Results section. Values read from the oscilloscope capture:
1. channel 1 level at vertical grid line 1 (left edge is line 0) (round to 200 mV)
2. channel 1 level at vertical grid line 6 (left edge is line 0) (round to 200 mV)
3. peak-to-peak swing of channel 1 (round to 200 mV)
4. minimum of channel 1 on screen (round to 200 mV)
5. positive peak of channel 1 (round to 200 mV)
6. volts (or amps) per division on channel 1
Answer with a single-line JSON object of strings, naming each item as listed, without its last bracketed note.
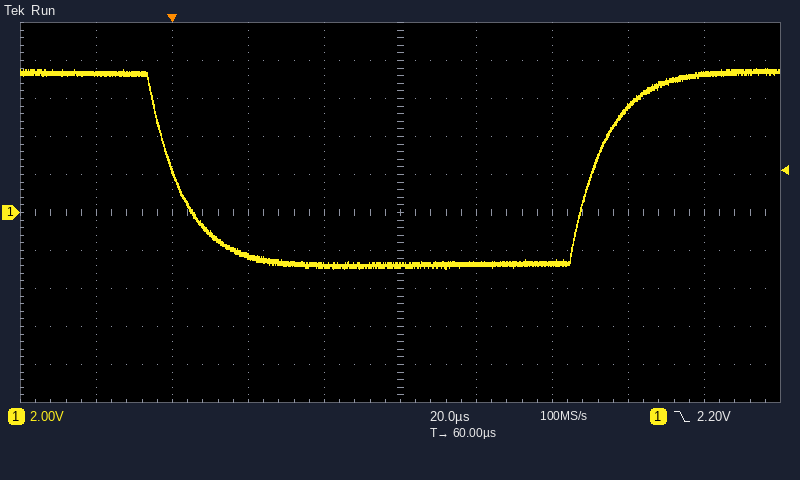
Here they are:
{"channel 1 level at vertical grid line 1 (left edge is line 0)": "7.4 V", "channel 1 level at vertical grid line 6 (left edge is line 0)": "-2.6 V", "peak-to-peak swing of channel 1": "10.6 V", "minimum of channel 1 on screen": "-3.0 V", "positive peak of channel 1": "7.6 V", "volts (or amps) per division on channel 1": "2 V"}
